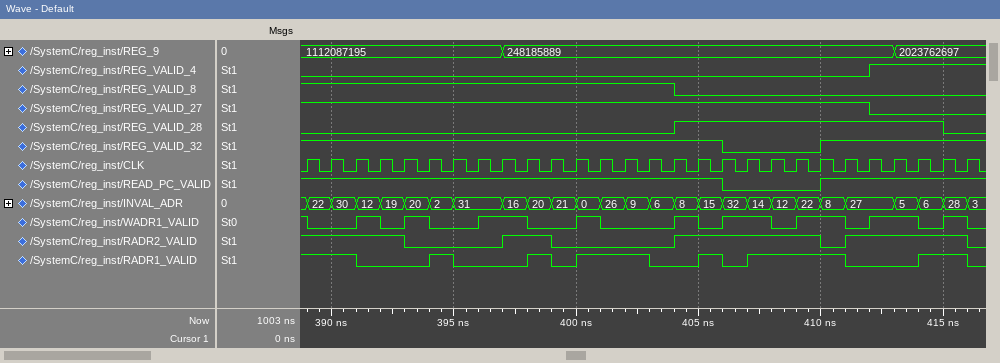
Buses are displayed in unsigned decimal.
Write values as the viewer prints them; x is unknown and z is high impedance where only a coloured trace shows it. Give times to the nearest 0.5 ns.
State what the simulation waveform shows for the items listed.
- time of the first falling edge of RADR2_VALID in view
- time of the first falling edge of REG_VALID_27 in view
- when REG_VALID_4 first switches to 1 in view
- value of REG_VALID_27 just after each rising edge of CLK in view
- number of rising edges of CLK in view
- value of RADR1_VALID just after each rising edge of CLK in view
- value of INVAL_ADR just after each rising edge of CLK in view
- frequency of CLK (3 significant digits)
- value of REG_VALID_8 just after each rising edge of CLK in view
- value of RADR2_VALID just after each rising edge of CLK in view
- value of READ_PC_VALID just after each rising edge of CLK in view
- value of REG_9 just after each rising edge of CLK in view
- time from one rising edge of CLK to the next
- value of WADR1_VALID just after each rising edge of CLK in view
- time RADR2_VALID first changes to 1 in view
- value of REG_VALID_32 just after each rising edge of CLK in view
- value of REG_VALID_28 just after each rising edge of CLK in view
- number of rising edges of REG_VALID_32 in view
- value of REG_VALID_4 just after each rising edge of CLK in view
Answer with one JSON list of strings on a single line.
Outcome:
["393 ns", "412 ns", "412 ns", "1 1 1 1 1 1 1 1 1 1 1 1 1 1 1 1 1 1 1 1 1 1 1 0 0 0 0 0", "28", "1 1 0 0 0 1 0 0 0 1 0 1 1 1 0 0 1 0 1 1 1 1 0 0 0 1 1 0", "22, 30, 12, 19, 20, 2, 31, 31, 16, 20, 21, 0, 26, 9, 6, 8, 15, 32, 14, 12, 22, 8, 27, 27, 5, 6, 28, 3", "1.00 GHz", "1 1 1 1 1 1 1 1 1 1 1 1 1 1 1 0 0 0 0 0 0 0 0 0 0 0 0 0", "1 1 1 1 0 0 0 0 1 1 0 0 0 0 0 1 1 1 1 1 1 0 1 1 1 1 1 0", "1 1 1 1 1 1 1 1 1 1 1 1 1 1 1 1 1 0 0 0 0 1 1 1 1 1 1 1", "1112087195, 1112087195, 1112087195, 1112087195, 1112087195, 1112087195, 1112087195, 1112087195, 248185889, 248185889, 248185889, 248185889, 248185889, 248185889, 248185889, 248185889, 248185889, 248185889, 248185889, 248185889, 248185889, 248185889, 248185889, 248185889, 2023762697, 2023762697, 2023762697, 2023762697", "1 ns", "0 0 1 0 1 0 0 1 1 0 0 1 0 0 0 1 0 1 1 0 1 1 0 1 1 0 1 0", "397 ns", "1 1 1 1 1 1 1 1 1 1 1 1 1 1 1 1 1 0 0 0 0 1 1 1 1 1 1 1", "0 0 0 0 0 0 0 0 0 0 0 0 0 0 0 1 1 1 1 1 1 1 1 1 1 1 0 0", "1", "0 0 0 0 0 0 0 0 0 0 0 0 0 0 0 0 0 0 0 0 0 0 0 1 1 1 1 1"]
